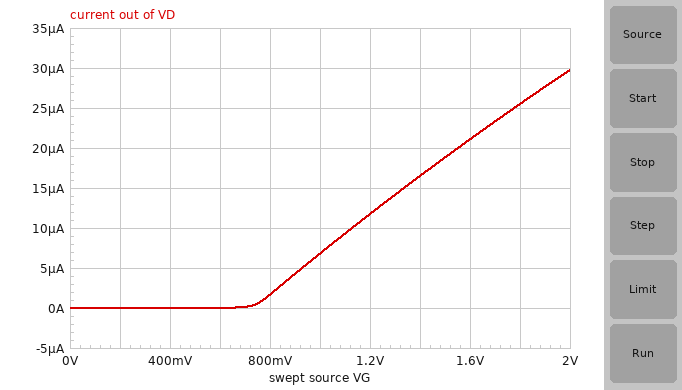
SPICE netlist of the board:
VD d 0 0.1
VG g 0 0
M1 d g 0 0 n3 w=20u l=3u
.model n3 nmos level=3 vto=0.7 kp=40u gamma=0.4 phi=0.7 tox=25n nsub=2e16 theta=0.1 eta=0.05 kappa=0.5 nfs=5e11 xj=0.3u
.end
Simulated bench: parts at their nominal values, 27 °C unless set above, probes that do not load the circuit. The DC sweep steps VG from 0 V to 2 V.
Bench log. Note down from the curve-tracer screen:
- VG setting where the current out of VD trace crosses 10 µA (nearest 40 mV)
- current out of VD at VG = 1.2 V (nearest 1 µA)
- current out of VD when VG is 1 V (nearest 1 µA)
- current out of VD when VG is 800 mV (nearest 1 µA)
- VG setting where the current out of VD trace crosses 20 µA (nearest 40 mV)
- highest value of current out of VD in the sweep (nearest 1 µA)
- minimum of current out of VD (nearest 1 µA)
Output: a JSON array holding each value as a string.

["1.12 V", "12 µA", "7 µA", "2 µA", "1.56 V", "30 µA", "0 A"]
